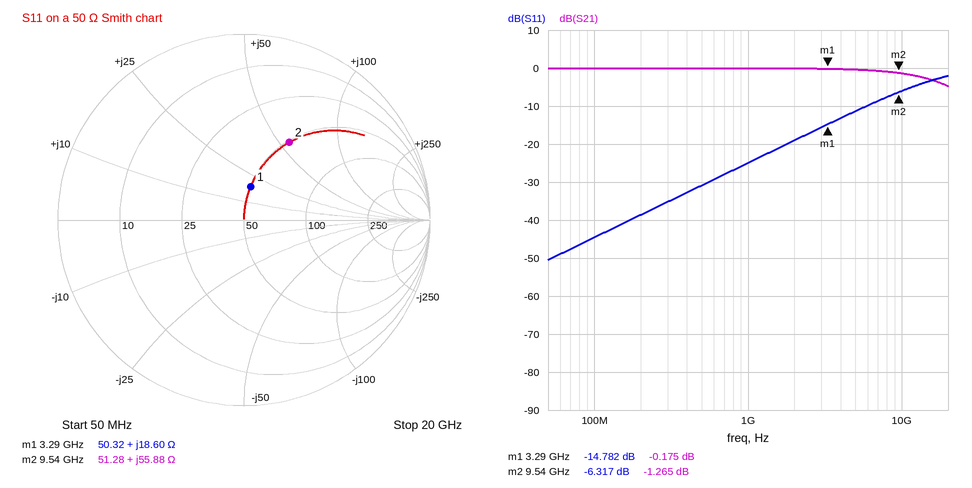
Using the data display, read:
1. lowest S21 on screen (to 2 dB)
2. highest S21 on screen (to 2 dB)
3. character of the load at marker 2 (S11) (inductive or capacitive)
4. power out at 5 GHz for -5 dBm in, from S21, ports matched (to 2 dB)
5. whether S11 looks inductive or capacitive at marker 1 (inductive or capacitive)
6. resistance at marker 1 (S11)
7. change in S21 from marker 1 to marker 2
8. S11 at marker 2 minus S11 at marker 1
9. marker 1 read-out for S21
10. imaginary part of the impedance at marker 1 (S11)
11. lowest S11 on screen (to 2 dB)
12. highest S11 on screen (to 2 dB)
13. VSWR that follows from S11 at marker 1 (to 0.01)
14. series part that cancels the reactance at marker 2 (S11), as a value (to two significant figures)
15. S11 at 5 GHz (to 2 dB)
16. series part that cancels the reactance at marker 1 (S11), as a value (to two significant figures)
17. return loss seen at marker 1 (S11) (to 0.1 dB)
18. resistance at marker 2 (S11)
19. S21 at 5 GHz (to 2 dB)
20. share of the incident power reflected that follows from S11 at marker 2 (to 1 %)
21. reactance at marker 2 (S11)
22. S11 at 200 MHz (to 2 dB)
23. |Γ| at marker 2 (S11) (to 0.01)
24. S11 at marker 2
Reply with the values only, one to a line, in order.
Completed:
-4 dB
0 dB
inductive
-6 dBm
inductive
50.32 Ω
-1.090 dB
8.465 dB
-0.175 dB
+18.60 Ω
-50 dB
-2 dB
1.45
300 fF
-12 dB
2.6 pF
14.8 dB
51.28 Ω
0 dB
23 %
+55.88 Ω
-38 dB
0.48
-6.317 dB
